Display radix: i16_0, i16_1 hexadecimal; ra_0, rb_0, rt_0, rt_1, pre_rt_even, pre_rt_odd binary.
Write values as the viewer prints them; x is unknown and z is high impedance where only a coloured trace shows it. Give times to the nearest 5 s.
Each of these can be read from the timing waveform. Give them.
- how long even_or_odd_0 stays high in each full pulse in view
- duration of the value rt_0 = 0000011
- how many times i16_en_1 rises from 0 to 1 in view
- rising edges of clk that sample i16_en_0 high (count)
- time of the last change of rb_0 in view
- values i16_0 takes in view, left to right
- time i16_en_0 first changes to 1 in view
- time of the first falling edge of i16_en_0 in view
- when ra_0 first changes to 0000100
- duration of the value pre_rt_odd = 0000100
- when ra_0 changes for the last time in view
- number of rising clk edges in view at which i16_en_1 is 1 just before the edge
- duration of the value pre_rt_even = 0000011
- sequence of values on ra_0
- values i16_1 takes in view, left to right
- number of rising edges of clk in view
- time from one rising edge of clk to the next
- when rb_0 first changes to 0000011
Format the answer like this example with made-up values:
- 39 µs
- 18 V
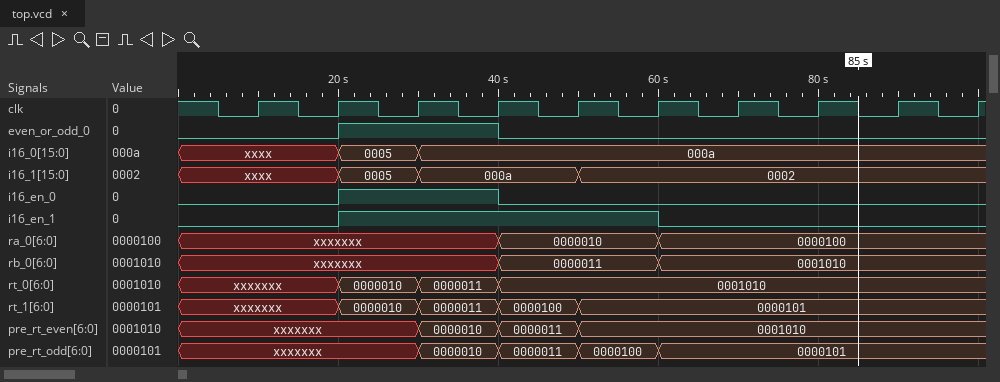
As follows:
- 20 s
- 10 s
- 1
- 2
- 60 s
- xxxx, 0005, 000a
- 20 s
- 40 s
- 60 s
- 10 s
- 60 s
- 4
- 10 s
- xxxxxxx, 0000010, 0000100
- xxxx, 0005, 000a, 0002
- 10
- 10 s
- 40 s
